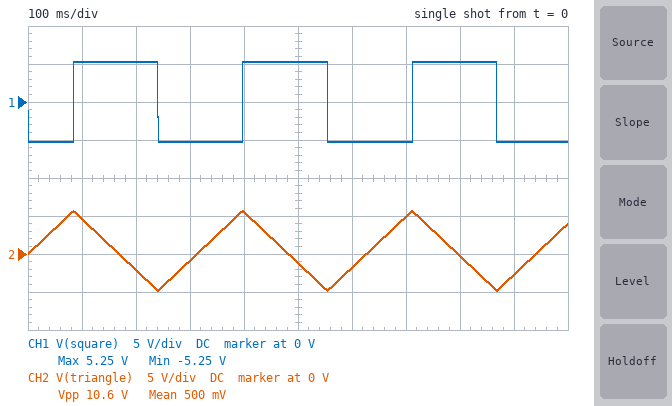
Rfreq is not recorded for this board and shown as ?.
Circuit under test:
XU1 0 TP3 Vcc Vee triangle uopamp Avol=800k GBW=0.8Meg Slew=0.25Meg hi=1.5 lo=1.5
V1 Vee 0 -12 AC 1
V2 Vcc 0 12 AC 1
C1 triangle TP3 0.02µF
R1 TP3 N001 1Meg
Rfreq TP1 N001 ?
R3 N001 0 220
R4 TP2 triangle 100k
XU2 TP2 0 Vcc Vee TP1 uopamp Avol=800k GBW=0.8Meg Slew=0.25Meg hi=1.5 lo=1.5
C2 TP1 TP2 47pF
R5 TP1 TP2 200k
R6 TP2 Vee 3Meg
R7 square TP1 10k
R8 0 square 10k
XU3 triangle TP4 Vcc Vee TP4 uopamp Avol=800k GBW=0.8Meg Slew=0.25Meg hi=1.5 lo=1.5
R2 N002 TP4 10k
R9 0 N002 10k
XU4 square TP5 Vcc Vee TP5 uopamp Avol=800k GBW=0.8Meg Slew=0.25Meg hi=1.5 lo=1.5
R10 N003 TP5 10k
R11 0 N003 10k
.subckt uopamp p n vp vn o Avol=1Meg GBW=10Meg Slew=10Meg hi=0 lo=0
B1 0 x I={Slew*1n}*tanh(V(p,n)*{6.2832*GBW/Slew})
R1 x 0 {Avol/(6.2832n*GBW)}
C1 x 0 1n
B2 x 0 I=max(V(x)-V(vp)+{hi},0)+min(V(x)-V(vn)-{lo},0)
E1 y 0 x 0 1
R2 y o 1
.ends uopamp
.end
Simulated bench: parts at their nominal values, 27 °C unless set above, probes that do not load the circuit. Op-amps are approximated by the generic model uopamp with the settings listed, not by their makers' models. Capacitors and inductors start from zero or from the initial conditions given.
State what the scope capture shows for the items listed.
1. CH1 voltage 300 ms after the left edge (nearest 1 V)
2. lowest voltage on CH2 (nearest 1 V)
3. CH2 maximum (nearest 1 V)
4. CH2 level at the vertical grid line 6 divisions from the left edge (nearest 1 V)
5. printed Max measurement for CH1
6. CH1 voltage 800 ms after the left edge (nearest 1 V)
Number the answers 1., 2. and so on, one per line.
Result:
1. -5 V
2. -5 V
3. 6 V
4. -2 V
5. 5.25 V
6. 5 V
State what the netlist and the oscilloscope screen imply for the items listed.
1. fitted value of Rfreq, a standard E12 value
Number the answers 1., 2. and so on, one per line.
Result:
1. 1.5 kΩ
